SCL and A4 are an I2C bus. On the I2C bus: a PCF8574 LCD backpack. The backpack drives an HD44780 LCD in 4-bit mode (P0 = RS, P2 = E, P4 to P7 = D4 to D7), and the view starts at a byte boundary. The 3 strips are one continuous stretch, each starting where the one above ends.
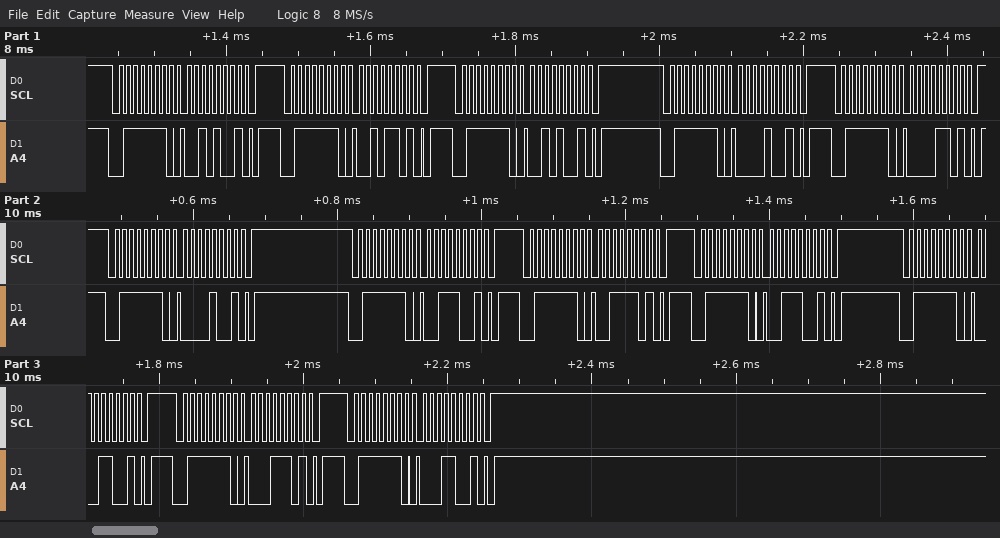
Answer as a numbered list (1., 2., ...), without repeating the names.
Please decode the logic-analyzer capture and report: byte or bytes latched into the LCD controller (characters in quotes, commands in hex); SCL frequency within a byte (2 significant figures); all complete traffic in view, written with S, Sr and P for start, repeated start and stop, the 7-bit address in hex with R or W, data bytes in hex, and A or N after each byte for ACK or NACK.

1. ' ' '1'
2. 100 kHz
3. S 3FW A 29 A P S 3FW A 2D A P S 3FW A 29 A P S 3FW A 09 A P S 3FW A 0D A P S 3FW A 09 A P S 3FW A 39 A P S 3FW A 3D A P S 3FW A 39 A P S 3FW A 19 A P S 3FW A 1D A P S 3FW A 19 A P
